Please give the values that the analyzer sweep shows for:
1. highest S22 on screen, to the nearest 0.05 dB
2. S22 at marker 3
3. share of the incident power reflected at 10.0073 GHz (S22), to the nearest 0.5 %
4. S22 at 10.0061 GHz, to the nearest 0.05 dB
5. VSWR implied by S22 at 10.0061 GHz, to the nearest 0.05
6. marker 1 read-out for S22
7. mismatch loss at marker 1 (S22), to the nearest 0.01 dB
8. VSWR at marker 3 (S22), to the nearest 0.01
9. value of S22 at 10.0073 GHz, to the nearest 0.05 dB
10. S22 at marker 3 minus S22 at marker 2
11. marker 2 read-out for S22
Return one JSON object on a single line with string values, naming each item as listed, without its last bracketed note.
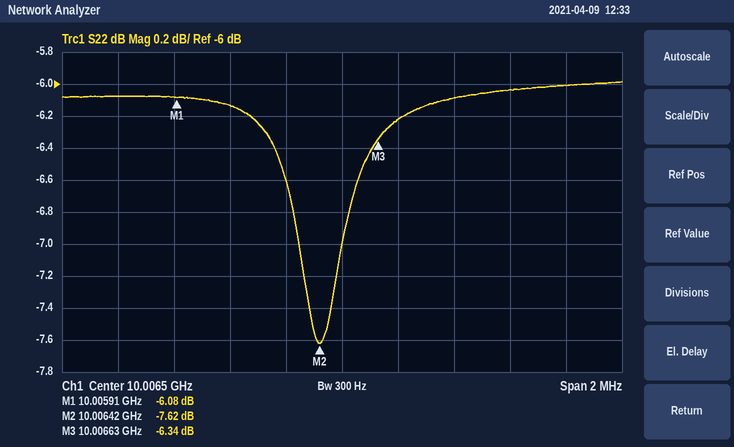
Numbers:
{"highest S22 on screen, to the nearest 0.05 dB": "-6.00 dB", "S22 at marker 3": "-6.34 dB", "share of the incident power reflected at 10.0073 GHz (S22), to the nearest 0.5 %": "25.0 %", "S22 at 10.0061 GHz, to the nearest 0.05 dB": "-6.15 dB", "VSWR implied by S22 at 10.0061 GHz, to the nearest 0.05": "2.95", "marker 1 read-out for S22": "-6.08 dB", "mismatch loss at marker 1 (S22), to the nearest 0.01 dB": "1.23 dB", "VSWR at marker 3 (S22), to the nearest 0.01": "2.86", "value of S22 at 10.0073 GHz, to the nearest 0.05 dB": "-6.00 dB", "S22 at marker 3 minus S22 at marker 2": "1.28 dB", "marker 2 read-out for S22": "-7.62 dB"}
